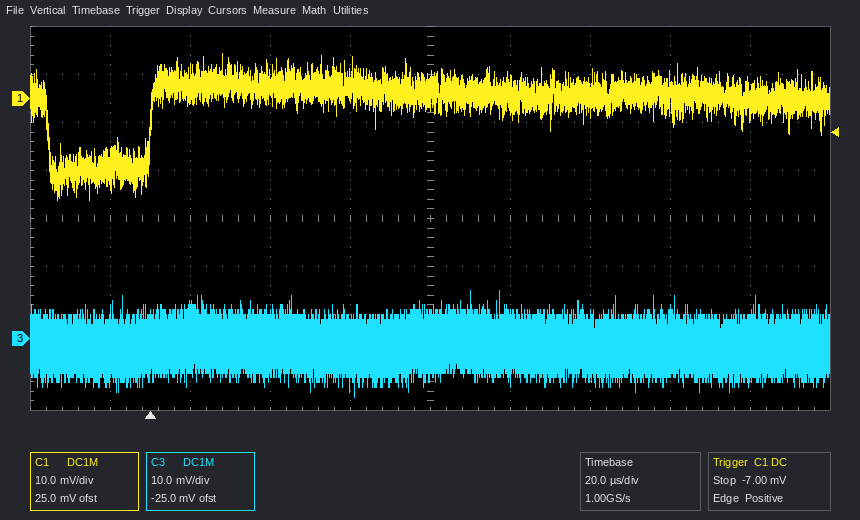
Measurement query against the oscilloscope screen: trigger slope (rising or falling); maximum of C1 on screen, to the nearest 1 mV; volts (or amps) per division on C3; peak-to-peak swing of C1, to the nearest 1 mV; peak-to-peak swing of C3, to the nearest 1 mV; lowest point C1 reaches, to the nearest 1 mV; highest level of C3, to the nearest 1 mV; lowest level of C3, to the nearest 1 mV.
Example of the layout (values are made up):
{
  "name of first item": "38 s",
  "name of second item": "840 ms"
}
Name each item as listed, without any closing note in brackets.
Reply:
{
  "trigger slope": "rising",
  "maximum of C1 on screen, to the nearest 1 mV": "9 mV",
  "volts (or amps) per division on C3": "10 mV",
  "peak-to-peak swing of C1, to the nearest 1 mV": "30 mV",
  "peak-to-peak swing of C3, to the nearest 1 mV": "22 mV",
  "lowest point C1 reaches, to the nearest 1 mV": "-21 mV",
  "highest level of C3, to the nearest 1 mV": "10 mV",
  "lowest level of C3, to the nearest 1 mV": "-12 mV"
}
